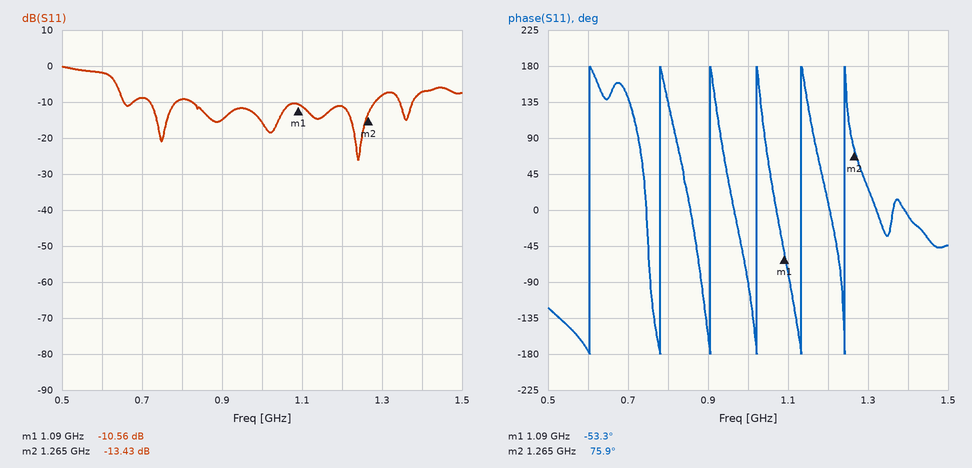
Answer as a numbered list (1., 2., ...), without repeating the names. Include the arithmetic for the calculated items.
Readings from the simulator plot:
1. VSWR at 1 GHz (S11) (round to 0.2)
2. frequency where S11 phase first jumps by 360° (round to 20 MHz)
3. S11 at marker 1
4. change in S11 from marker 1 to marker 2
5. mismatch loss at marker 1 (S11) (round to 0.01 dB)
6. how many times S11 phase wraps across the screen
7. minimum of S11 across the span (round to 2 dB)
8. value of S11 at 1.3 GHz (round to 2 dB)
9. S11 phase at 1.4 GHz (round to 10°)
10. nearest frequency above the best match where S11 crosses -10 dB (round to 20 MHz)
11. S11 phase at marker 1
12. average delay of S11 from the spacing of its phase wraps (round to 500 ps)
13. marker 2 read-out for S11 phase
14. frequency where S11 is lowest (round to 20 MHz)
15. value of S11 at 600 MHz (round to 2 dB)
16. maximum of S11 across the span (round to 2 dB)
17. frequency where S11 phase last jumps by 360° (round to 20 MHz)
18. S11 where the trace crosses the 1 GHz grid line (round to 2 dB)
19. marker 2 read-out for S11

1. |Γ| = 10^(-16/20) = 0.1585; VSWR = (1 + 0.1585)/(1 − 0.1585) ≈ 1.4
2. 600 MHz
3. -10.56 dB
4. -13.43 − (-10.56) = -2.87 dB
5. −10 log10(1 − 10^(-10.56/10)) ≈ 0.40 dB
6. 6
7. -26 dB
8. -8 dB
9. -10°
10. 1.28 GHz
11. -53.3°
12. 5 cycles / (1.24 GHz − 600 MHz) ≈ 7.81 ns, so 8.0 ns to the nearest 500 ps
13. 75.9°
14. 1.24 GHz
15. -2 dB
16. 0 dB
17. 1.24 GHz
18. -16 dB
19. -13.43 dB
